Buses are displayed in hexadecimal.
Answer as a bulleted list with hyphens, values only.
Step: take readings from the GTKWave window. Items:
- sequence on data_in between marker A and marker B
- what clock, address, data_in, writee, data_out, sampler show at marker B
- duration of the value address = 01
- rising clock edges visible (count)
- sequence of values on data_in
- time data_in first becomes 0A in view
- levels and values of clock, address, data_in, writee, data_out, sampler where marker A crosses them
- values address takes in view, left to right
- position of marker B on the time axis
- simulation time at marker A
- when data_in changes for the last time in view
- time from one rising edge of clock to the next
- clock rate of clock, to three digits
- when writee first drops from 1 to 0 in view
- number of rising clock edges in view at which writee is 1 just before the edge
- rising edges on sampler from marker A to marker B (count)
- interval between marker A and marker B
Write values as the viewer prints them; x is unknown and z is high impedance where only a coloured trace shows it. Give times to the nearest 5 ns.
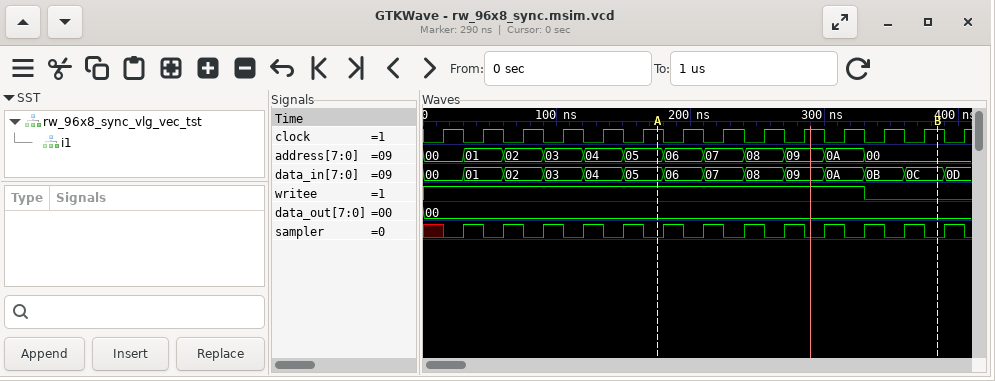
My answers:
- 05, 06, 07, 08, 09, 0A, 0B, 0C
- clock=1, address=00, data_in=0C, writee=0, data_out=00, sampler=0
- 30 ns
- 14
- 00, 01, 02, 03, 04, 05, 06, 07, 08, 09, 0A, 0B, 0C, 0D
- 300 ns
- clock=1, address=05, data_in=05, writee=1, data_out=00, sampler=0
- 00, 01, 02, 03, 04, 05, 06, 07, 08, 09, 0A, 00
- 385 ns
- 175 ns
- 390 ns
- 30 ns
- 33.3 MHz
- 330 ns
- 11
- 7
- 210 ns
